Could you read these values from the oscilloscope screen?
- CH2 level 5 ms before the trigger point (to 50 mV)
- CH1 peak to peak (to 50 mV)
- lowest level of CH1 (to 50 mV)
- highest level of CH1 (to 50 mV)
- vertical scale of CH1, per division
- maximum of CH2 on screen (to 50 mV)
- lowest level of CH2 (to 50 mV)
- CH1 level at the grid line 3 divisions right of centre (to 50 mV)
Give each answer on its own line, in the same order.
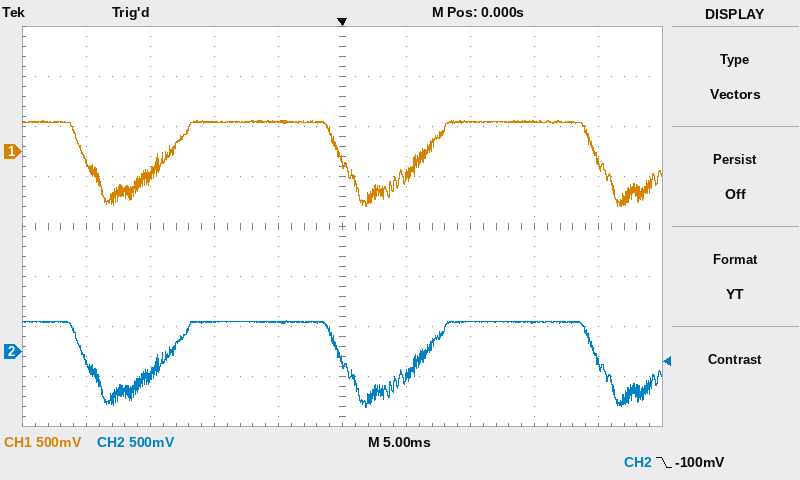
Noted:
300 mV
850 mV
-550 mV
300 mV
500 mV
300 mV
-550 mV
300 mV
